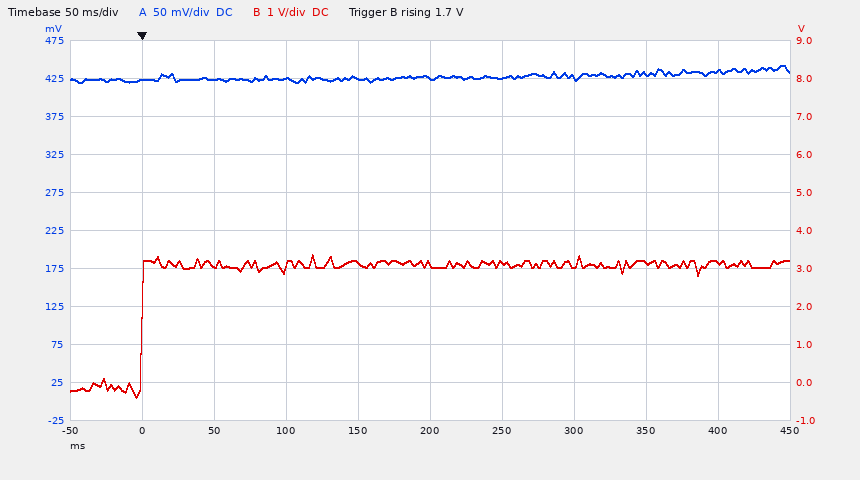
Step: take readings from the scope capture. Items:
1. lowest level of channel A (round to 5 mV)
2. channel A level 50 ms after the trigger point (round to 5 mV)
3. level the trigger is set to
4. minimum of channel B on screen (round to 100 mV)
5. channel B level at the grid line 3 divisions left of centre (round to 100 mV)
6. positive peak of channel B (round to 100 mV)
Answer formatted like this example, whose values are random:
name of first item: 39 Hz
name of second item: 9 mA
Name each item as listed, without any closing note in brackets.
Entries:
lowest level of channel A: 420 mV
channel A level 50 ms after the trigger point: 425 mV
level the trigger is set to: 1.7 V
minimum of channel B on screen: -400 mV
channel B level at the grid line 3 divisions left of centre: 3.1 V
positive peak of channel B: 3.4 V
